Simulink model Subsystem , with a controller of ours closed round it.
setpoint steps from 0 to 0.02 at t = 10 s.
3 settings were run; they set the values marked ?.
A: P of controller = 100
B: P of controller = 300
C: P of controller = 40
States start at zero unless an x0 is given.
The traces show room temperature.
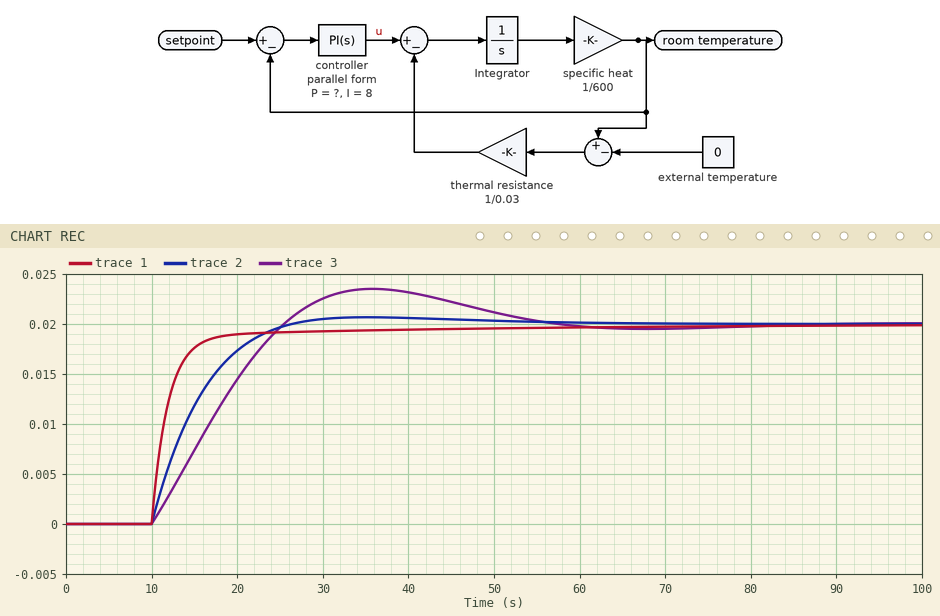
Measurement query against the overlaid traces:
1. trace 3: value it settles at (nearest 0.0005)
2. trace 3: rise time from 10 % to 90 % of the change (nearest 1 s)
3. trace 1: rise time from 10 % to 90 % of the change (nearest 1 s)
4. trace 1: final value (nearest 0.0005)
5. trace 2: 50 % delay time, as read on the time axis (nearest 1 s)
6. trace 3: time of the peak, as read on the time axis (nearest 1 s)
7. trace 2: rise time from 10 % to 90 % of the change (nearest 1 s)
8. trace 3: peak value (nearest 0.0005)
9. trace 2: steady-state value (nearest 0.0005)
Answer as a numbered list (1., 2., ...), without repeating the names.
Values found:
1. 0.0200
2. 12 s
3. 5 s
4. 0.0200
5. 14 s
6. 36 s
7. 10 s
8. 0.0235
9. 0.0200
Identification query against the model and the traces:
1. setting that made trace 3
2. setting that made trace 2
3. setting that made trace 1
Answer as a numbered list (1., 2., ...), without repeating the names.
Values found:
1. C
2. A
3. B
